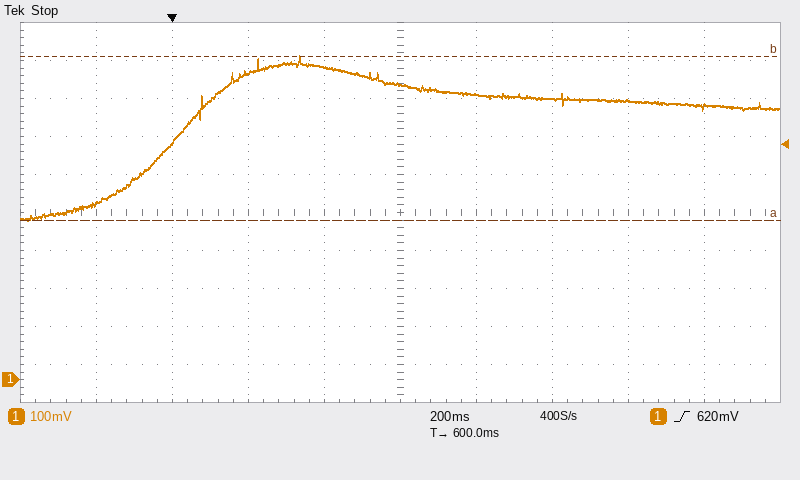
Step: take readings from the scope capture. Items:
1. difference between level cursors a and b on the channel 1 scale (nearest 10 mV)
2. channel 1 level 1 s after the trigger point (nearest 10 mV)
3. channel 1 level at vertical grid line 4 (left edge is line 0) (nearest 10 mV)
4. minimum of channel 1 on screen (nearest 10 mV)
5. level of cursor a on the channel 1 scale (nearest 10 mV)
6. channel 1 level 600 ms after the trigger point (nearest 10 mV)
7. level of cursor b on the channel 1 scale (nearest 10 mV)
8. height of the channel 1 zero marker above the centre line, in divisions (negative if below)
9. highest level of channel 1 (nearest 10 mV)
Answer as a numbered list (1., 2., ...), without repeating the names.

1. 430 mV
2. 740 mV
3. 820 mV
4. 420 mV
5. 420 mV
6. 780 mV
7. 850 mV
8. -4.4 div
9. 850 mV
